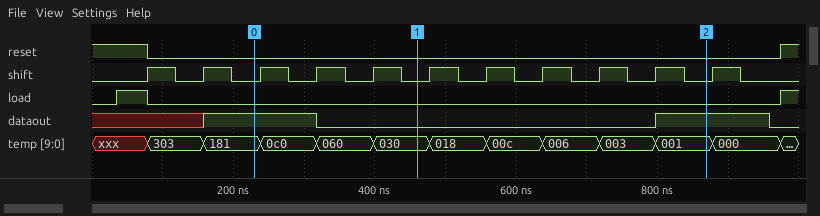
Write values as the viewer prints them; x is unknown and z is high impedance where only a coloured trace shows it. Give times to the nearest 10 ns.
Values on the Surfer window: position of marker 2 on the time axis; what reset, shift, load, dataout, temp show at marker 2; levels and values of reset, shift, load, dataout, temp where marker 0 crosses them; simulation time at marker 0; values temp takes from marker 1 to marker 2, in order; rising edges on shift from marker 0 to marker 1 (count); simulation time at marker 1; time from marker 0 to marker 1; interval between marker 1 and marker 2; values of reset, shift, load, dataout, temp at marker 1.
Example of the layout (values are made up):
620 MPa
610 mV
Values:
870 ns
reset=0, shift=0, load=0, dataout=1, temp=001
reset=0, shift=0, load=0, dataout=1, temp=181
230 ns
030, 018, 00c, 006, 003, 001
3
460 ns
230 ns
410 ns
reset=0, shift=0, load=0, dataout=0, temp=030
